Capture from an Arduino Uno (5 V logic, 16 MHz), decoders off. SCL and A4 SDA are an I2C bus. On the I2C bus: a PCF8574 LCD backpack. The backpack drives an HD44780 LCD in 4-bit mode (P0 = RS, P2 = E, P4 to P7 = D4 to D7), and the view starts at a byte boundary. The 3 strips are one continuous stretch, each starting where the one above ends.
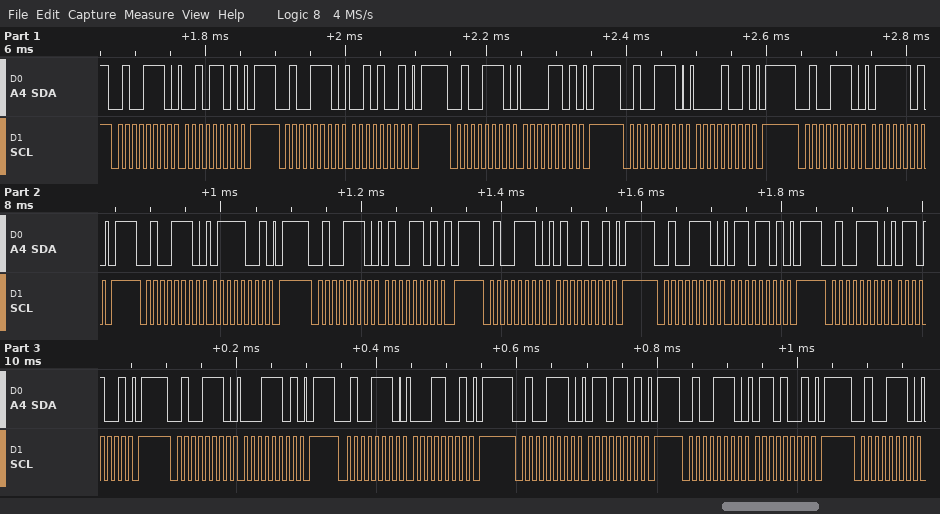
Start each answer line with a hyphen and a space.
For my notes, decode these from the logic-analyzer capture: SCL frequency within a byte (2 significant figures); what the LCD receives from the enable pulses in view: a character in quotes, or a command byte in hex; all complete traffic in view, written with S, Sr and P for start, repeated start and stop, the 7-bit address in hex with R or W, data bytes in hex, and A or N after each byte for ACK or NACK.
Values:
- 100 kHz
- ' ' 't' 'a'
- S 27W A 2D A P S 27W A 29 A P S 27W A 0D A P S 27W A 09 A P S 27W A 7D A P S 27W A 79 A P S 27W A 4D A P S 27W A 49 A P S 27W A 6D A P S 27W A 69 A P S 27W A 1D A P S 27W A 19 A P S 27W A 6D A P S 27W A 69 A P S 27W A
